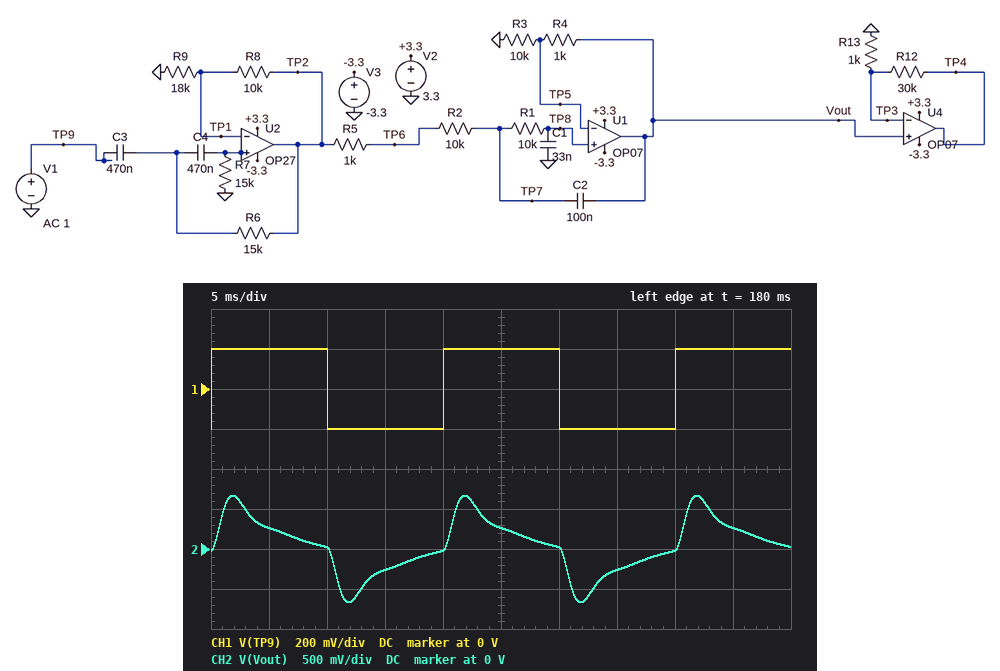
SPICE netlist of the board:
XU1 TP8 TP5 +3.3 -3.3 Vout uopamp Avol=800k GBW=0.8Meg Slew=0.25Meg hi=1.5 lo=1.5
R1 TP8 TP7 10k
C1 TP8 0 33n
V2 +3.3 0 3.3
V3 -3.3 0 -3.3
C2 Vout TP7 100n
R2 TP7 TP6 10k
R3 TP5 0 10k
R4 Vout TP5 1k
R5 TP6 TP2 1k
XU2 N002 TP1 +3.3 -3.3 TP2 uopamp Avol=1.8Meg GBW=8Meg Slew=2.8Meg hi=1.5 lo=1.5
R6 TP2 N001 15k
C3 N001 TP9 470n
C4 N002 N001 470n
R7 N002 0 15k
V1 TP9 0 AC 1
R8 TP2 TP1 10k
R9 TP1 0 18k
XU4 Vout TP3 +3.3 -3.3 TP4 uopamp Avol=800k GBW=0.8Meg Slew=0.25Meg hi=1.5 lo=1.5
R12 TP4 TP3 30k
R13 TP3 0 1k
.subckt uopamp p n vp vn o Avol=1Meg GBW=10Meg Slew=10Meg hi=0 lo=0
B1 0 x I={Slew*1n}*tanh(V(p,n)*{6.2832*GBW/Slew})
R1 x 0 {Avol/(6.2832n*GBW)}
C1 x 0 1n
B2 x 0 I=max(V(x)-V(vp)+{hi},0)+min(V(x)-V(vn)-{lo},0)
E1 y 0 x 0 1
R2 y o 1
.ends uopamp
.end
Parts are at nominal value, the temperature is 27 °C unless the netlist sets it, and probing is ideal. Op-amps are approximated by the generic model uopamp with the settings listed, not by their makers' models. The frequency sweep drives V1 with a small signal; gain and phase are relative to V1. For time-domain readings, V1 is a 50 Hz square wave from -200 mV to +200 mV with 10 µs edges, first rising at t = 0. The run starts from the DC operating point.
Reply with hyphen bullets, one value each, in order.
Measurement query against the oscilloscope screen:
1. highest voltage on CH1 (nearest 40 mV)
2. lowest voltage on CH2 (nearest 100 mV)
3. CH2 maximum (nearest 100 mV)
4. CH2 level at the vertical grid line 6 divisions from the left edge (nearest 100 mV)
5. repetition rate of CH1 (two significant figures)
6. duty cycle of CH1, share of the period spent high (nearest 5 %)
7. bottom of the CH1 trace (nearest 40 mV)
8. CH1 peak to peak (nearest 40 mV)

- 200 mV
- -700 mV
- 700 mV
- 0 V
- 50 Hz
- 50 %
- -200 mV
- 400 mV
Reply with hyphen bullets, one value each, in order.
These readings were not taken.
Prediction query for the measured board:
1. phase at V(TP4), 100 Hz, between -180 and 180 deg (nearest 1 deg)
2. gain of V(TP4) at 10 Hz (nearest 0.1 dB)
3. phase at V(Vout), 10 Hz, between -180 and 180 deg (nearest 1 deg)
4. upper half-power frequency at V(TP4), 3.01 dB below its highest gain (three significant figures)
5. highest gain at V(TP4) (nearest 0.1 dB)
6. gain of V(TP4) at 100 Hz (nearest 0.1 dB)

- -4 deg
- 20.1 dB
- 139 deg
- 310 Hz
- 35.9 dB
- 35.1 dB
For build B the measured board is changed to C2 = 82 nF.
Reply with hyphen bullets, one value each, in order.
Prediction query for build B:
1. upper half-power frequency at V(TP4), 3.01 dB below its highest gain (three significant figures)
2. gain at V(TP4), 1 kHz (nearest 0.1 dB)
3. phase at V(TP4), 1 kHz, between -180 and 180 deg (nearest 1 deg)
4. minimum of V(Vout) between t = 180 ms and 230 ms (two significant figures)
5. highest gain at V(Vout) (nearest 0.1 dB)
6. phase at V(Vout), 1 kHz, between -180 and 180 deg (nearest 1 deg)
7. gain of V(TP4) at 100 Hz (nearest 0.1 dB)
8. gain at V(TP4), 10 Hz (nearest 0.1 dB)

- 334 Hz
- 13.3 dB
- -161 deg
- -640 mV
- 5.4 dB
- -159 deg
- 34.8 dB
- 20.1 dB
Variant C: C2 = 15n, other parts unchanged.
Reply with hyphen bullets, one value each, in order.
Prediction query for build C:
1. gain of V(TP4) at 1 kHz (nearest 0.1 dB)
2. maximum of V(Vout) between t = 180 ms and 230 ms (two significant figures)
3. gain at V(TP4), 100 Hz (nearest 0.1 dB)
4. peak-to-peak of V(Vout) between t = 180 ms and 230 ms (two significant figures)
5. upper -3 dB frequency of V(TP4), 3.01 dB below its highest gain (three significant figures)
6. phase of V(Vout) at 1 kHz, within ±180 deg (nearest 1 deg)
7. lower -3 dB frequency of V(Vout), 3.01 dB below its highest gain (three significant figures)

- 21.6 dB
- 520 mV
- 33.9 dB
- 1.0 V
- 287 Hz
- -103 deg
- 22.2 Hz
